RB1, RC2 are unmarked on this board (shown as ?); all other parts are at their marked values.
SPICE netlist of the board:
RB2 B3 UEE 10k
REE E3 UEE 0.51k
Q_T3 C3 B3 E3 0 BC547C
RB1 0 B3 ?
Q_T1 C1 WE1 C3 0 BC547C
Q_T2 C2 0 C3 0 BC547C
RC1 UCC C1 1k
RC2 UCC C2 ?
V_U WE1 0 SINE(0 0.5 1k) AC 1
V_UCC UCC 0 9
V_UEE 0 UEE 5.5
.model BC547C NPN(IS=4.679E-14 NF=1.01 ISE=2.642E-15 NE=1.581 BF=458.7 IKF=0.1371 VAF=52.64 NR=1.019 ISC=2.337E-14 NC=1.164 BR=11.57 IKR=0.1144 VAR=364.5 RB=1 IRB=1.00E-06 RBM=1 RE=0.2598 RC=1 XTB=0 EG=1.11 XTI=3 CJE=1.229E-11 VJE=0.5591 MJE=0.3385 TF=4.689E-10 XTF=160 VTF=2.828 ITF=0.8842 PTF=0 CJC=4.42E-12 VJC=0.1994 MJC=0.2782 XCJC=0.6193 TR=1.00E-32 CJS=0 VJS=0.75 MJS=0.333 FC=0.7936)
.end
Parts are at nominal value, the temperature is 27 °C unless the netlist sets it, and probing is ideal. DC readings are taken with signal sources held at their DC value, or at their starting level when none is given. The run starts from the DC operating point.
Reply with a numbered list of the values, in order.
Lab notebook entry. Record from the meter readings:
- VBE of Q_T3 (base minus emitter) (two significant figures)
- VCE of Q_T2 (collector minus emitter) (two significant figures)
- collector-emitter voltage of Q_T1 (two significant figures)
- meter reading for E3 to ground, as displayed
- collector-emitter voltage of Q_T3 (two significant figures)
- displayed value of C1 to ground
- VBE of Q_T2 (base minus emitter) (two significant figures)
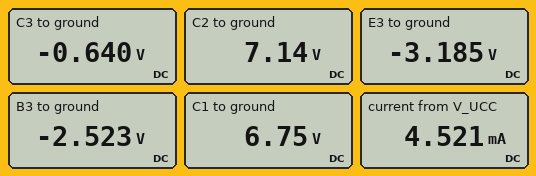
1. 660 mV
2. 7.8 V
3. 7.4 V
4. -3.185 V
5. 2.5 V
6. 6.75 V
7. 640 mV
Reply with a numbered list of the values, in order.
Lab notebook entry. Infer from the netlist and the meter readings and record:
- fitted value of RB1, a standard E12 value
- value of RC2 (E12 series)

1. 8.2 kΩ
2. 820 Ω
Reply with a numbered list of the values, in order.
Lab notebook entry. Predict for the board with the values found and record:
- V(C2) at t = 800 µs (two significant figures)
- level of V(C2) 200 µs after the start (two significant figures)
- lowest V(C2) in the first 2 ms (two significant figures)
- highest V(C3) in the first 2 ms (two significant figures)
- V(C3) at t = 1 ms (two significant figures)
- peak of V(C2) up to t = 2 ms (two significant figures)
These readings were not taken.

1. 5.3 V
2. 9.0 V
3. 5.3 V
4. -160 mV
5. -640 mV
6. 9.0 V
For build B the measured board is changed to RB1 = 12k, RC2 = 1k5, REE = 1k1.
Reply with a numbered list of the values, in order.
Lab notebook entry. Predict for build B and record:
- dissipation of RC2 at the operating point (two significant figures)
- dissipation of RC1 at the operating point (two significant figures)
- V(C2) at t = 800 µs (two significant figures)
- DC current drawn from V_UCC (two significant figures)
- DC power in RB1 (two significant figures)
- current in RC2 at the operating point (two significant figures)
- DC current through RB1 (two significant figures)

1. 1.0 mW
2. 700 µW
3. 6.5 V
4. 1.7 mA
5. 760 µW
6. 830 µA
7. 250 µA
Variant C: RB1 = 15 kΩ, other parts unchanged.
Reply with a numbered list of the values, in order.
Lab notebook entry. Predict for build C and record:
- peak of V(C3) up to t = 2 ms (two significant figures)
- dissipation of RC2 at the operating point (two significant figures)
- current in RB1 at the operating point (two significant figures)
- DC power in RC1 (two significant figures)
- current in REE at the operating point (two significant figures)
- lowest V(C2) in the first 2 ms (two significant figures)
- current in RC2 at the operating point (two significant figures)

1. -150 mV
2. 1.8 mW
3. 220 µA
4. 2.2 mW
5. 3.0 mA
6. 6.6 V
7. 1.5 mA
